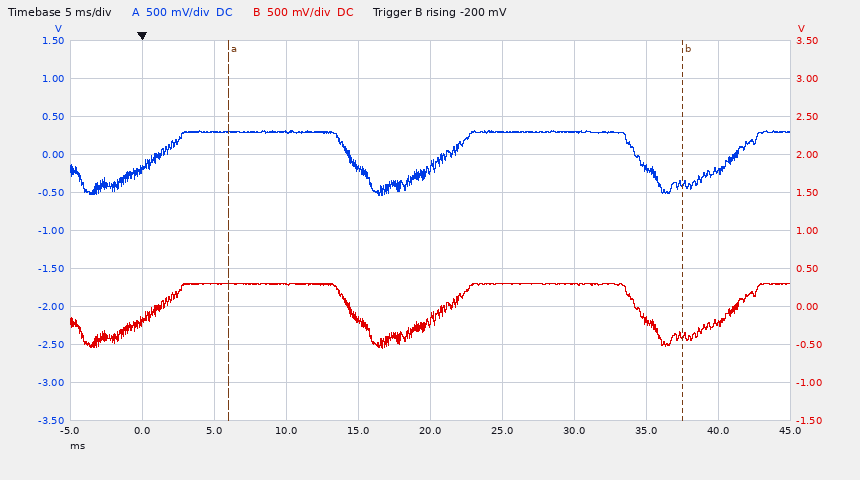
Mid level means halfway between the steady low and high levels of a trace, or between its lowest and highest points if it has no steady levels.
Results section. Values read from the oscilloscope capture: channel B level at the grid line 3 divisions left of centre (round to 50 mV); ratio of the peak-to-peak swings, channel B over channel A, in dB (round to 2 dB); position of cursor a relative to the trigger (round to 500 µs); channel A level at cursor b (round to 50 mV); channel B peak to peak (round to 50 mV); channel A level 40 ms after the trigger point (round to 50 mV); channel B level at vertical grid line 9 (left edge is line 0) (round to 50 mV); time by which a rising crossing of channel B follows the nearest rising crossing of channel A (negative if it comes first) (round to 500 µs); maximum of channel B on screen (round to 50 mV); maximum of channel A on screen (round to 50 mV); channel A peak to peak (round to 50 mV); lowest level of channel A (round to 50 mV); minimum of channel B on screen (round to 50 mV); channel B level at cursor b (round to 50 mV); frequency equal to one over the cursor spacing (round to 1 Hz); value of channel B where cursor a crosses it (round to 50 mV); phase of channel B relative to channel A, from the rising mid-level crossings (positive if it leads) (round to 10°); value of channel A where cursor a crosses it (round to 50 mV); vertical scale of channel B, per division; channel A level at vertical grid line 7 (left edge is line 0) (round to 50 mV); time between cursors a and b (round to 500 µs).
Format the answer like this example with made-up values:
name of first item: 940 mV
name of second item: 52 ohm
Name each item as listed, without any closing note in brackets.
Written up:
channel B level at the grid line 3 divisions left of centre: 300 mV
ratio of the peak-to-peak swings, channel B over channel A, in dB: 0 dB
position of cursor a relative to the trigger: +6.0 ms
channel A level at cursor b: -400 mV
channel B peak to peak: 850 mV
channel A level 40 ms after the trigger point: -200 mV
channel B level at vertical grid line 9 (left edge is line 0): -200 mV
time by which a rising crossing of channel B follows the nearest rising crossing of channel A (negative if it comes first): 0.0 ms
maximum of channel B on screen: 300 mV
maximum of channel A on screen: 300 mV
channel A peak to peak: 850 mV
lowest level of channel A: -550 mV
minimum of channel B on screen: -550 mV
channel B level at cursor b: -400 mV
frequency equal to one over the cursor spacing: 32 Hz
value of channel B where cursor a crosses it: 300 mV
phase of channel B relative to channel A, from the rising mid-level crossings (positive if it leads): 0°
value of channel A where cursor a crosses it: 300 mV
vertical scale of channel B, per division: 500 mV
channel A level at vertical grid line 7 (left edge is line 0): 300 mV
time between cursors a and b: 31.5 ms
